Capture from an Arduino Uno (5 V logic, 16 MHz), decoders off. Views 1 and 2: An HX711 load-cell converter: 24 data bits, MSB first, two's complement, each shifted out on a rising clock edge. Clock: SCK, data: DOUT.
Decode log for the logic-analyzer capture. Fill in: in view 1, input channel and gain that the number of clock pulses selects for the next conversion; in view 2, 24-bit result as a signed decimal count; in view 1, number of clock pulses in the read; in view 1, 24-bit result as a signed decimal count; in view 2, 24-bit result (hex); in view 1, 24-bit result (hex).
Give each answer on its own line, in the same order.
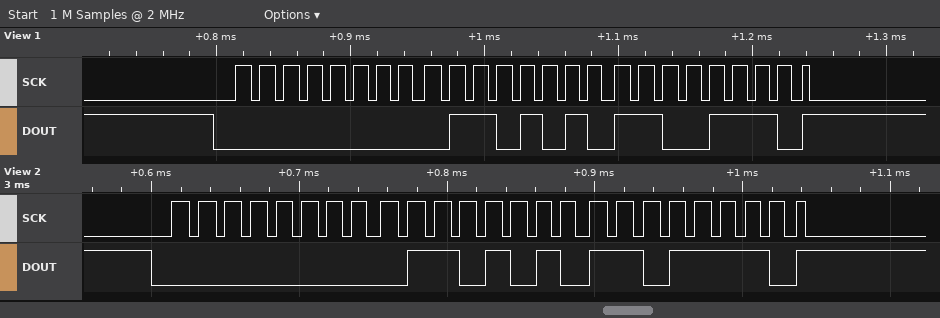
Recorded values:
channel A, gain 128
27358
25
27342
0x006ADE
0x006ACE
